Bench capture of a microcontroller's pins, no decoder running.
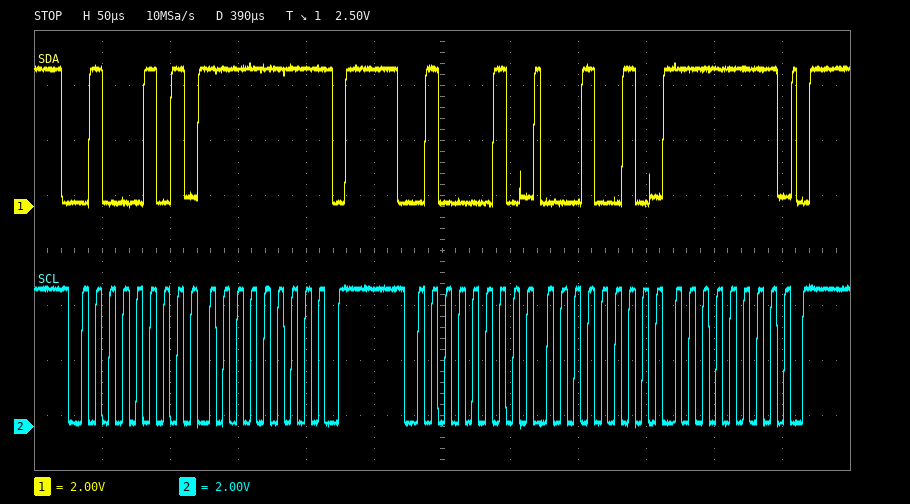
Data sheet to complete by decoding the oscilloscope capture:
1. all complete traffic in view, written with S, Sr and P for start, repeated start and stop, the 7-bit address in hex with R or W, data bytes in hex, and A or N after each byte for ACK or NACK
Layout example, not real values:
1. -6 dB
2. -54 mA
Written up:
1. S 22R A FF N P S 21W A 12 A FF A P
